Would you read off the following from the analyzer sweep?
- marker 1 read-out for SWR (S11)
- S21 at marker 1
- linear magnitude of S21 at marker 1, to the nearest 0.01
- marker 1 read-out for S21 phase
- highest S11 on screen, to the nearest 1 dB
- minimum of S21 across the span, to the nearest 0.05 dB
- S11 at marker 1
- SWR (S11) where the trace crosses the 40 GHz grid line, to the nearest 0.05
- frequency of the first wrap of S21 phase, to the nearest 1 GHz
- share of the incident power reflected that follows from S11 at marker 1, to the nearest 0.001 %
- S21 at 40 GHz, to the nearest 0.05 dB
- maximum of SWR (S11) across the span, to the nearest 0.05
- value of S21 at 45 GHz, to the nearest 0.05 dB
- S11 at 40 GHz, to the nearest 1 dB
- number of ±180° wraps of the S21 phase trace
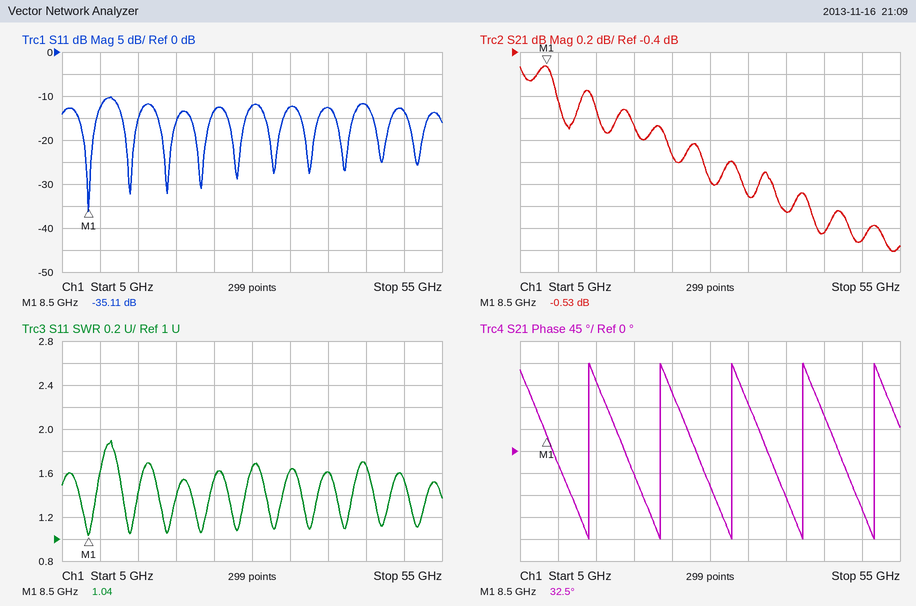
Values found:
1.04
-0.53 dB
0.94
32.5°
-10 dB
-2.20 dB
-35.11 dB
1.60
14 GHz
0.031 %
-1.85 dB
1.90
-2.05 dB
-13 dB
5
